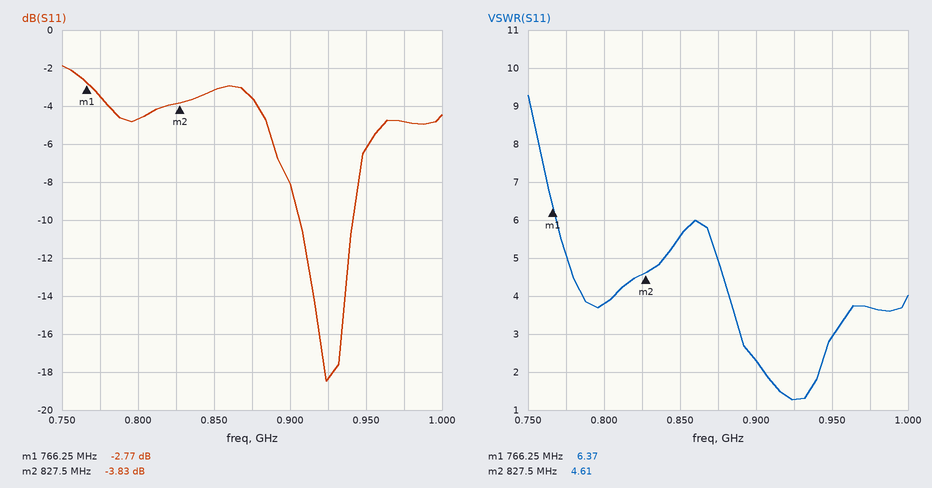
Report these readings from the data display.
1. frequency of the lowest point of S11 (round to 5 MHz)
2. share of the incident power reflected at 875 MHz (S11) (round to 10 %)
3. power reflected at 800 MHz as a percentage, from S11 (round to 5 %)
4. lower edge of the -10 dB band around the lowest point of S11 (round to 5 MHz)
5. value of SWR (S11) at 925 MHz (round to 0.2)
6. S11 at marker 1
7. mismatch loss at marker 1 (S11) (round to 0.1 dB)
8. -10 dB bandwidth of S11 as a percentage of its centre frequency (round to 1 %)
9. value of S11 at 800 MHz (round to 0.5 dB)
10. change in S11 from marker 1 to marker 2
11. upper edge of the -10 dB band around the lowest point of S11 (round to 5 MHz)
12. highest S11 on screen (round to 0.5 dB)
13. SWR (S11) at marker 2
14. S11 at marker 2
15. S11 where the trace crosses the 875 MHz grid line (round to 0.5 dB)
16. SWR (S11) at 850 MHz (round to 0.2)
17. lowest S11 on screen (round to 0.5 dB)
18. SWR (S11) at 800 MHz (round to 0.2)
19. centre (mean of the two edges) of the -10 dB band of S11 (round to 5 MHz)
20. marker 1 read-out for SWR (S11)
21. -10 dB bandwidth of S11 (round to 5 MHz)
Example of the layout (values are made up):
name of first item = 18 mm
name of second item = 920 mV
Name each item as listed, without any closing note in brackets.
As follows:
frequency of the lowest point of S11 = 925 MHz
share of the incident power reflected at 875 MHz (S11) = 40 %
power reflected at 800 MHz as a percentage, from S11 = 35 %
lower edge of the -10 dB band around the lowest point of S11 = 905 MHz
value of SWR (S11) at 925 MHz = 1.2
S11 at marker 1 = -2.77 dB
mismatch loss at marker 1 (S11) = 3.3 dB
-10 dB bandwidth of S11 as a percentage of its centre frequency = 4 %
value of S11 at 800 MHz = -4.5 dB
change in S11 from marker 1 to marker 2 = -1.06 dB
upper edge of the -10 dB band around the lowest point of S11 = 940 MHz
highest S11 on screen = -2.0 dB
SWR (S11) at marker 2 = 4.61
S11 at marker 2 = -3.83 dB
S11 where the trace crosses the 875 MHz grid line = -3.5 dB
SWR (S11) at 850 MHz = 5.6
lowest S11 on screen = -18.5 dB
SWR (S11) at 800 MHz = 3.8
centre (mean of the two edges) of the -10 dB band of S11 = 925 MHz
marker 1 read-out for SWR = 6.37
-10 dB bandwidth of S11 = 35 MHz
